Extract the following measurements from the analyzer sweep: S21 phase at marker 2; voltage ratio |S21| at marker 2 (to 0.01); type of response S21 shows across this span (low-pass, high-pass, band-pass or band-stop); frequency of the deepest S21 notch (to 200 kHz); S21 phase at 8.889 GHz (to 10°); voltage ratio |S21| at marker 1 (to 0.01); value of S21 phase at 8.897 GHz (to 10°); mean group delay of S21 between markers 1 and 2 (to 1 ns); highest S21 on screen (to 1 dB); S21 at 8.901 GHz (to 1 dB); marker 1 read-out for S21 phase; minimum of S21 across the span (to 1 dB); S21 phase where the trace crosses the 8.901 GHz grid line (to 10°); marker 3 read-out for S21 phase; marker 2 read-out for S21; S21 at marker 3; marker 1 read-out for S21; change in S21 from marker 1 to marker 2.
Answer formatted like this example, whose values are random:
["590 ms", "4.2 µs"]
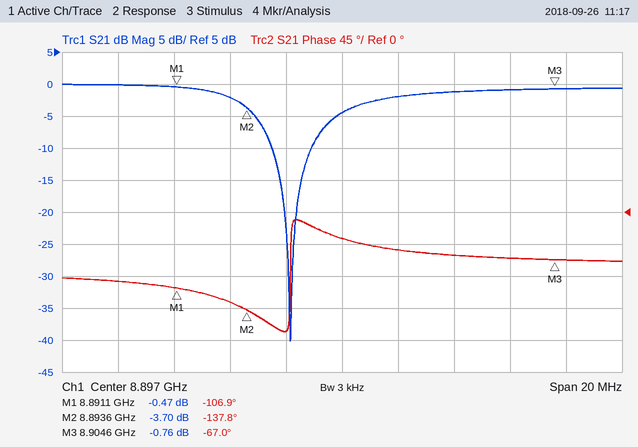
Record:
["-137.8°", "0.65", "band-stop", "8.8952 GHz", "-100°", "0.95", "-40°", "34 ns", "0 dB", "-1 dB", "-106.9°", "-40 dB", "-60°", "-67.0°", "-3.70 dB", "-0.76 dB", "-0.47 dB", "-3.23 dB"]
